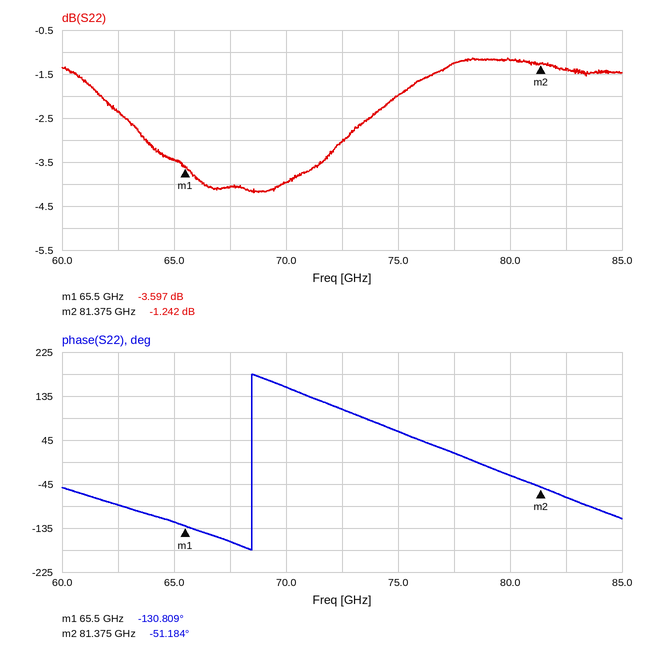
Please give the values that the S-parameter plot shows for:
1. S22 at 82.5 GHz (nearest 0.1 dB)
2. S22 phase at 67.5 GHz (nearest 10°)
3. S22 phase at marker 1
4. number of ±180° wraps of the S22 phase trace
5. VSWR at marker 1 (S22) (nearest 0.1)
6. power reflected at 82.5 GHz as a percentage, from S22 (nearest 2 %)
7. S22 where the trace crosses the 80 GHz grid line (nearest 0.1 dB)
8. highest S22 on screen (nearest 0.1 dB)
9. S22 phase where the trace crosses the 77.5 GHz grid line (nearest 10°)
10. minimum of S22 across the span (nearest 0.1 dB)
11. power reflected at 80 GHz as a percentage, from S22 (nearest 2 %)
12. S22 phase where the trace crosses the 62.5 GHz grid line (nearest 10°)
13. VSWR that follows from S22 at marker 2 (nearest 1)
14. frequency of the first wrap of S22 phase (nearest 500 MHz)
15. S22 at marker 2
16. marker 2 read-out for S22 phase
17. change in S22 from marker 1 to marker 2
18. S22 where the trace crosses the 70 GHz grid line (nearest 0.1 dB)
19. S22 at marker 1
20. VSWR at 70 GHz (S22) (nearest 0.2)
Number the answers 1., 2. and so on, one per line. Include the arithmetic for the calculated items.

1. -1.4 dB
2. -160°
3. -130.809°
4. 1
5. (1 + 0.6609)/(1 − 0.6609) ≈ 4.9
6. 10^(-1.4/10) ≈ 72 %
7. -1.2 dB
8. -1.1 dB
9. 20°
10. -4.2 dB
11. 10^(-1.2/10) ≈ 76 %
12. -90°
13. (1 + 0.8668)/(1 − 0.8668) ≈ 14
14. 68.5 GHz
15. -1.242 dB
16. -51.184°
17. -1.242 − (-3.597) = 2.355 dB
18. -4.0 dB
19. -3.597 dB
20. |Γ| = 10^(-4/20) = 0.6310; VSWR = (1 + 0.6310)/(1 − 0.6310) ≈ 4.4
